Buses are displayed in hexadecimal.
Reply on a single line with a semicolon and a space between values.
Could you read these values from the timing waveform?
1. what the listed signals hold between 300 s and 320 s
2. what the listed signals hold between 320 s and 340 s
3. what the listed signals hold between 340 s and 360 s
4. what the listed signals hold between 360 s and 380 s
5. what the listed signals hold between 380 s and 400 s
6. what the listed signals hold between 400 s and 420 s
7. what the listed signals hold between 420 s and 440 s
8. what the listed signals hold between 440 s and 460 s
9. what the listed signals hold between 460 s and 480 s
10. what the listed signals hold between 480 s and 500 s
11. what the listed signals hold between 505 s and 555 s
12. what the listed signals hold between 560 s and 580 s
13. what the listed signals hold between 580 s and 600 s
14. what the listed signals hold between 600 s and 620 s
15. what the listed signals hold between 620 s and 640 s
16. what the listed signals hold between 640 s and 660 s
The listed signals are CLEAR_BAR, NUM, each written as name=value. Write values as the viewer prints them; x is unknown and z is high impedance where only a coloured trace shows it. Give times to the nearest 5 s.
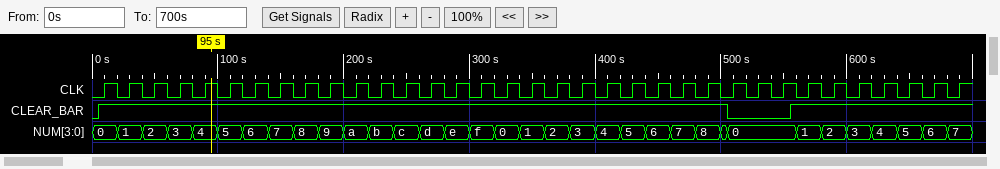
CLEAR_BAR=1, NUM=f; CLEAR_BAR=1, NUM=0; CLEAR_BAR=1, NUM=1; CLEAR_BAR=1, NUM=2; CLEAR_BAR=1, NUM=3; CLEAR_BAR=1, NUM=4; CLEAR_BAR=1, NUM=5; CLEAR_BAR=1, NUM=6; CLEAR_BAR=1, NUM=7; CLEAR_BAR=1, NUM=8; CLEAR_BAR=0, NUM=0; CLEAR_BAR=1, NUM=1; CLEAR_BAR=1, NUM=2; CLEAR_BAR=1, NUM=3; CLEAR_BAR=1, NUM=4; CLEAR_BAR=1, NUM=5
